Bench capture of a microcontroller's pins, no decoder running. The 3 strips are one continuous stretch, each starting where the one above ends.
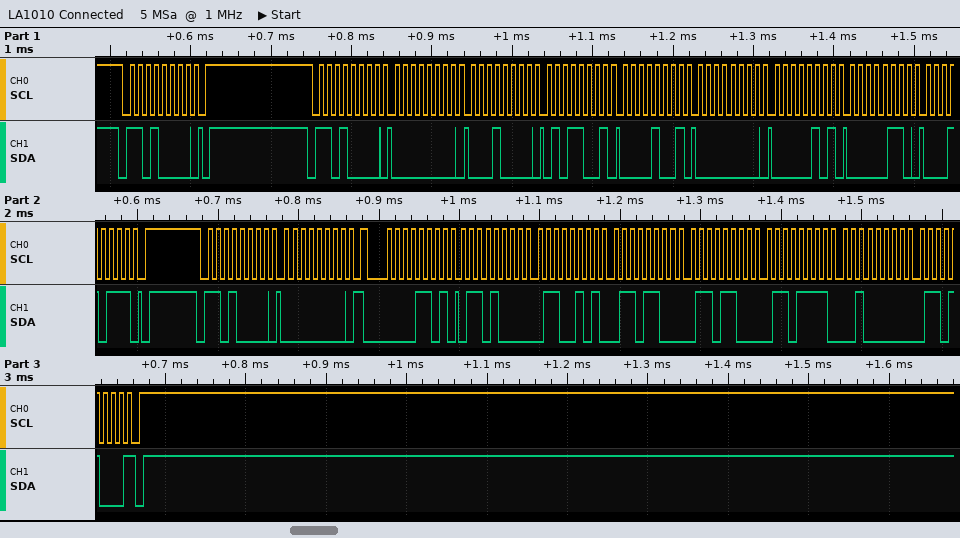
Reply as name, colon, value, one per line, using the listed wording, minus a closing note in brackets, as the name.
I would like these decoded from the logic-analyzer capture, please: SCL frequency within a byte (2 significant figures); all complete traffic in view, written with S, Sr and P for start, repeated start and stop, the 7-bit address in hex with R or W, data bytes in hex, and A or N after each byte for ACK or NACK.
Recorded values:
SCL frequency within a byte: 100 kHz
all complete traffic in view, written with S, Sr and P for start, repeated start and stop, the 7-bit address in hex with R or W, data bytes in hex, and A or N after each byte for ACK or NACK: S 68W A P S 68W A 00 A 10 A 59 A 09 A 00 A 05 A 06 A 17 A P S 68W A 00 A Sr 06R A 68 A 65 A 6C A 6C A 6F A 20 A 68 N P
